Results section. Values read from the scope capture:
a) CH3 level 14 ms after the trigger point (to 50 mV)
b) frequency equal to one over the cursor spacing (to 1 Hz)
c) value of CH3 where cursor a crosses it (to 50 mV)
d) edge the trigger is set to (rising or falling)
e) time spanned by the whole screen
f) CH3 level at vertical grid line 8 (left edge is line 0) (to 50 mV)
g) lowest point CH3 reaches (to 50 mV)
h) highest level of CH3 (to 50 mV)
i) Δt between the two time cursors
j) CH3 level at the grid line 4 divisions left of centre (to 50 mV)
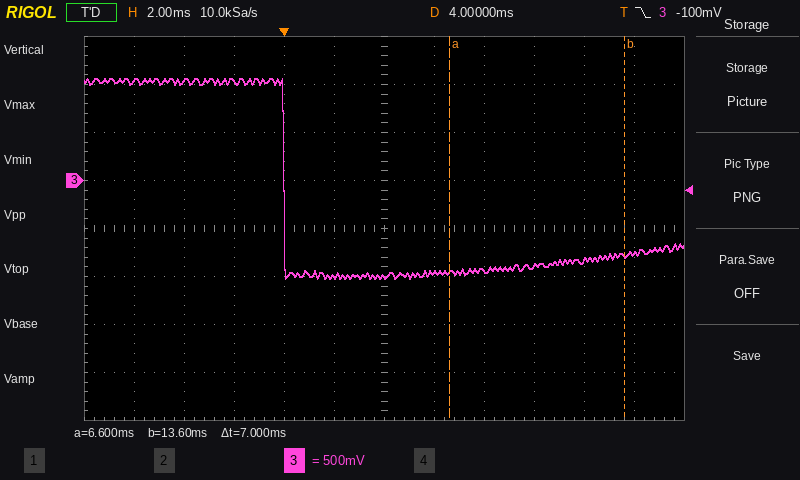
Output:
-750 mV
143 Hz
-950 mV
falling
24 ms
-950 mV
-1.00 V
1.05 V
7 ms
1.05 V
